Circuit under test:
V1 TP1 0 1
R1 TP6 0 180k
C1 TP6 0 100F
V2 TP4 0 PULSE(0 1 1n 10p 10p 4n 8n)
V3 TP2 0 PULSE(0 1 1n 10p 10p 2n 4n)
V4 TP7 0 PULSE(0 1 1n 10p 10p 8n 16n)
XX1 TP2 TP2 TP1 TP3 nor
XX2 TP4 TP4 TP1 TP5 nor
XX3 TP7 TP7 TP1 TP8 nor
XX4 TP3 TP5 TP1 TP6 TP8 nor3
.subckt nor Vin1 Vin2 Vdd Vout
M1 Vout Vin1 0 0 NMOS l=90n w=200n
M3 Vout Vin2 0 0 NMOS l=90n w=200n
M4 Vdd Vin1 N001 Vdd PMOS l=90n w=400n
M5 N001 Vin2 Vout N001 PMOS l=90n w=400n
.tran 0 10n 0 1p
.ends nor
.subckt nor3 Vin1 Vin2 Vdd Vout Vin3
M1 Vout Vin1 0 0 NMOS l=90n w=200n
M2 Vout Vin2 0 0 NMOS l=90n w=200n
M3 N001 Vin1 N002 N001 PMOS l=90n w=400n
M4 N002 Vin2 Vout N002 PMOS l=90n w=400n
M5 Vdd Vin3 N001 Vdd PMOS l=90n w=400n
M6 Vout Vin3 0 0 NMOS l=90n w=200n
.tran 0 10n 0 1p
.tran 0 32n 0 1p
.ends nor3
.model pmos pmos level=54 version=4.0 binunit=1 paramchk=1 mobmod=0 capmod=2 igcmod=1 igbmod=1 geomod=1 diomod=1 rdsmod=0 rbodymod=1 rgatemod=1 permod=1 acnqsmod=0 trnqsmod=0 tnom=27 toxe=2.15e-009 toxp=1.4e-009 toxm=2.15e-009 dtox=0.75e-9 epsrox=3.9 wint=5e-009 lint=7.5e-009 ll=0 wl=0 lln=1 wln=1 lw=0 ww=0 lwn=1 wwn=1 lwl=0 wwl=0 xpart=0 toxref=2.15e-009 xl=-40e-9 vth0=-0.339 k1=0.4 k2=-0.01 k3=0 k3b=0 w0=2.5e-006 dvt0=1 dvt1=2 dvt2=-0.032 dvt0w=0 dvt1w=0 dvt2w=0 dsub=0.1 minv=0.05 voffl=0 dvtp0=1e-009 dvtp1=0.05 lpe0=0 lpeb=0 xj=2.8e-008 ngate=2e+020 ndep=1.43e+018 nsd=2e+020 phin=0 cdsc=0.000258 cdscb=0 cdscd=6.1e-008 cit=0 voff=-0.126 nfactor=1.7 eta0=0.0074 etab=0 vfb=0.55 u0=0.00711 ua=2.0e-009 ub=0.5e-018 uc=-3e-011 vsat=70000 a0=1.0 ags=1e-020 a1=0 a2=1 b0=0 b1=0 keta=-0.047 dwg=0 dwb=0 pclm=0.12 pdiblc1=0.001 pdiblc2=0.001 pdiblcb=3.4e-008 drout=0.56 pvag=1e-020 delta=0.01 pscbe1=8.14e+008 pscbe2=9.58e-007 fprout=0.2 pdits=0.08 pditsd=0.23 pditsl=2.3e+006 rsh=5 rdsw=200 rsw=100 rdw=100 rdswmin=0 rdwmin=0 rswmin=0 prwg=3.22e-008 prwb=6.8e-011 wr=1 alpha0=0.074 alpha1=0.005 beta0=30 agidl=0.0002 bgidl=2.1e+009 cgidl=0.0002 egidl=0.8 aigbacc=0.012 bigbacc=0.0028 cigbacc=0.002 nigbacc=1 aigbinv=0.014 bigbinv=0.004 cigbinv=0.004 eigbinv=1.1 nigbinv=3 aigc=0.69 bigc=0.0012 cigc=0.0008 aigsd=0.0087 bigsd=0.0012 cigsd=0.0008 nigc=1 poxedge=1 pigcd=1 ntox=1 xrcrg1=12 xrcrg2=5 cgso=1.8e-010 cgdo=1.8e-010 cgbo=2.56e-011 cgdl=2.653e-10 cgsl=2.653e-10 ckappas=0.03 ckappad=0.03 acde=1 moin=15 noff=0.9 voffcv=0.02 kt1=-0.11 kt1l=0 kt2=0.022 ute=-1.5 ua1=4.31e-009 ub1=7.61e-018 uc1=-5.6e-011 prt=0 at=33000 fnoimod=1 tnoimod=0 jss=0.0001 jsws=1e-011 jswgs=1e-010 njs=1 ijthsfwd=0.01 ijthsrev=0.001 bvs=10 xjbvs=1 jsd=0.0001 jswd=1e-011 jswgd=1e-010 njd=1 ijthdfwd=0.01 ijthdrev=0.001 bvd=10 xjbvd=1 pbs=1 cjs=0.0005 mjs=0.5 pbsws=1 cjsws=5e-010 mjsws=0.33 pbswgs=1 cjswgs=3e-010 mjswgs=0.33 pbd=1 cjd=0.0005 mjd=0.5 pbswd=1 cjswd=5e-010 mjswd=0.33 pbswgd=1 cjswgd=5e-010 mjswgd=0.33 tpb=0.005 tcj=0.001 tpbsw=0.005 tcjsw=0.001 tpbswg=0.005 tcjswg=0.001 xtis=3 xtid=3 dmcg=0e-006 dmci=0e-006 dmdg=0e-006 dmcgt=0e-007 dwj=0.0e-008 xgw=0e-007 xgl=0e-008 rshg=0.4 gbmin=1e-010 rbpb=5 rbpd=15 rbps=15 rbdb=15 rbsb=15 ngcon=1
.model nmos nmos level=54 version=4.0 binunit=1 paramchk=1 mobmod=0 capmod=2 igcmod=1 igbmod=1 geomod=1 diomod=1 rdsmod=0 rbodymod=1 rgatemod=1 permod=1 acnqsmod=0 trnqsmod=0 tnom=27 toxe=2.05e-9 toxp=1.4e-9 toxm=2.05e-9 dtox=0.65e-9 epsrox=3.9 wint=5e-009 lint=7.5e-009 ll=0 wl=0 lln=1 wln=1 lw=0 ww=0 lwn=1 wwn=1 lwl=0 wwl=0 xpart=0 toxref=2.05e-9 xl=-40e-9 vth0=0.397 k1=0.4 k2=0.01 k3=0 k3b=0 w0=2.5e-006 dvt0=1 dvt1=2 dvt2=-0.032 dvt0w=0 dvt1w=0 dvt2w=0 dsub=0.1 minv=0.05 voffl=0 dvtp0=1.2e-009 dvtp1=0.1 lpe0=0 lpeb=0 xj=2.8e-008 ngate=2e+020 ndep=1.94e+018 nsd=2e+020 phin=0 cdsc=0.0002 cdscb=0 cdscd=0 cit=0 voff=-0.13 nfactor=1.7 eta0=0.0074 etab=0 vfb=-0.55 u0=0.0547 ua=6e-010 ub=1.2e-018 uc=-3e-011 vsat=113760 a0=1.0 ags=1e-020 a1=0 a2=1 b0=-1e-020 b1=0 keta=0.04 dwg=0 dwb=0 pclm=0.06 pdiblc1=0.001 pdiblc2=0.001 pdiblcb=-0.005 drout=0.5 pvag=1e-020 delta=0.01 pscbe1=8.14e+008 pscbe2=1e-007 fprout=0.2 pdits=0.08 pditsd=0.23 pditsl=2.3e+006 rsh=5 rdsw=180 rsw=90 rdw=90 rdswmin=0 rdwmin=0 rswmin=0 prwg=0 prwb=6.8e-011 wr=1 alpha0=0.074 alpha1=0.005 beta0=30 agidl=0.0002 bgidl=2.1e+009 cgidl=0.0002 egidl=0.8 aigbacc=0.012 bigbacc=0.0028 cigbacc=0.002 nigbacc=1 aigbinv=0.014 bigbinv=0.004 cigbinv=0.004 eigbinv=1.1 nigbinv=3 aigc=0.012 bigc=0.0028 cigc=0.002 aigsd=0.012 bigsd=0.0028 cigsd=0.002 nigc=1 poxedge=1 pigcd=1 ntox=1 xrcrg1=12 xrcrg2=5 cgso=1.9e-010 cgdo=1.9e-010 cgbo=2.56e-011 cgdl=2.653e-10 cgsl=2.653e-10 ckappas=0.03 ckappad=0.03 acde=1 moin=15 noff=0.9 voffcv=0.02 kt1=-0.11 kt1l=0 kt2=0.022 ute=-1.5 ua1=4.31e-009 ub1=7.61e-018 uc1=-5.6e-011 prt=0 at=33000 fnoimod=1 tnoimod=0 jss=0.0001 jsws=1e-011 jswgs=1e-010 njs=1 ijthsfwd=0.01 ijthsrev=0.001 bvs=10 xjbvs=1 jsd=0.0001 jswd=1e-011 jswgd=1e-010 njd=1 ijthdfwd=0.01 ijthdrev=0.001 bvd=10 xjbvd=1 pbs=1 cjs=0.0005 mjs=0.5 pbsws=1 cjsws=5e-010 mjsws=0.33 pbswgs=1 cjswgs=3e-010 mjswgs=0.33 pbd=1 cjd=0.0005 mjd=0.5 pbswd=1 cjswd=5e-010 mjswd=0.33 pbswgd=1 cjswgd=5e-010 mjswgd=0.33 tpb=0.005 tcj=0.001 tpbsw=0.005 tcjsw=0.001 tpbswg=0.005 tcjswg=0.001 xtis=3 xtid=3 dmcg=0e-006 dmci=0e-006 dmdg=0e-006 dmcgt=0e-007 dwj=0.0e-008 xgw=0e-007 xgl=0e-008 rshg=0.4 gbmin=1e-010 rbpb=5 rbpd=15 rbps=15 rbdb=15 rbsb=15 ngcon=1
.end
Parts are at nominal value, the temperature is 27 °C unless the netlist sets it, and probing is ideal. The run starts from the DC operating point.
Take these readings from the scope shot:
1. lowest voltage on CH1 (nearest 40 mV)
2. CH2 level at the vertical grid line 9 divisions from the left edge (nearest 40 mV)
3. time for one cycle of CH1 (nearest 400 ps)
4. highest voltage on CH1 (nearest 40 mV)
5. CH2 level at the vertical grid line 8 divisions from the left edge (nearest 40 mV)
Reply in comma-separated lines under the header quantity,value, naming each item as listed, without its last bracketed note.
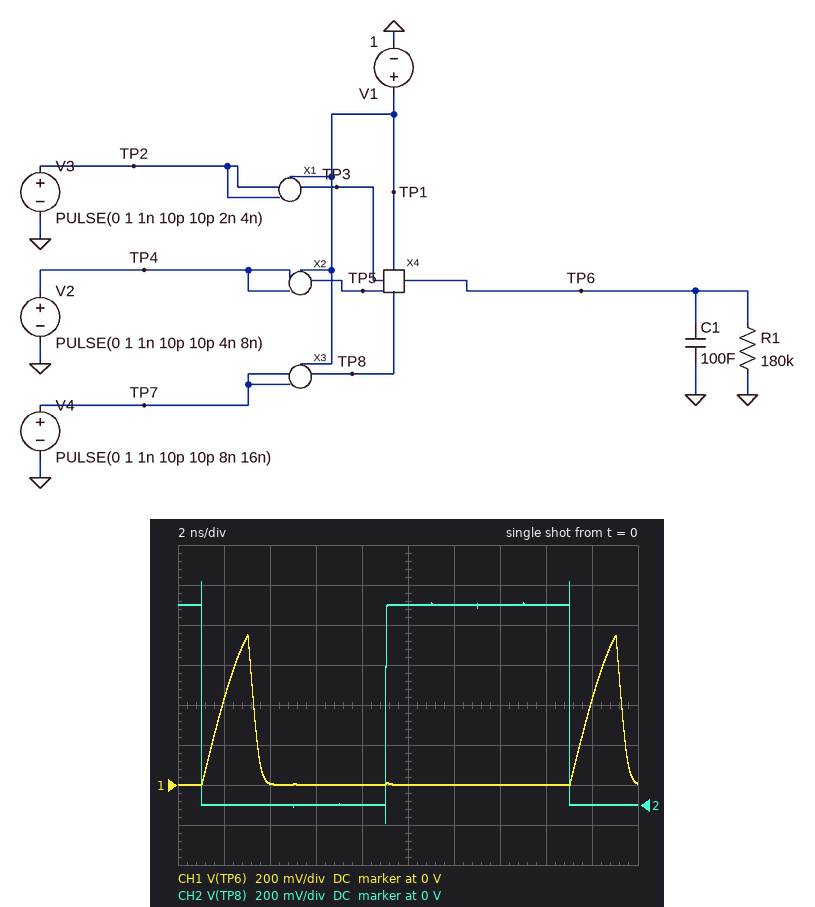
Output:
quantity,value
lowest voltage on CH1,0 V
CH2 level at the vertical grid line 9 divisions from the left edge,0 V
time for one cycle of CH1,16.0 ns
highest voltage on CH1,760 mV
CH2 level at the vertical grid line 8 divisions from the left edge,1.00 V
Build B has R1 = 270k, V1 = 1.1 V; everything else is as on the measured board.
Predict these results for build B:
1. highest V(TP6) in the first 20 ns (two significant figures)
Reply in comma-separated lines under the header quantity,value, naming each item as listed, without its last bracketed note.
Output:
quantity,value
highest V(TP6) in the first 20 ns,890 mV
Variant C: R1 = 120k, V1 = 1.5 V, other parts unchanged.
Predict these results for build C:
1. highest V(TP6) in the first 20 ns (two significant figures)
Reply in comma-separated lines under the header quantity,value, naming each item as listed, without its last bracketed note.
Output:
quantity,value
highest V(TP6) in the first 20 ns,1.3 V
